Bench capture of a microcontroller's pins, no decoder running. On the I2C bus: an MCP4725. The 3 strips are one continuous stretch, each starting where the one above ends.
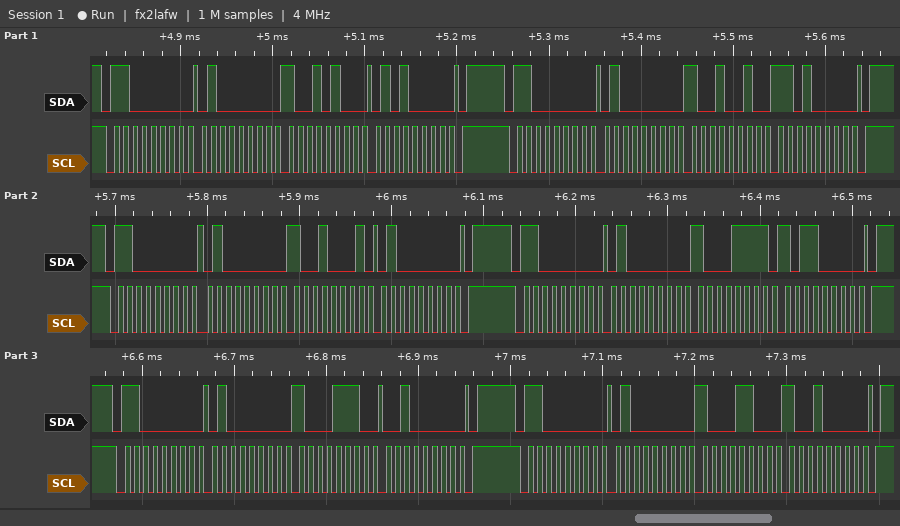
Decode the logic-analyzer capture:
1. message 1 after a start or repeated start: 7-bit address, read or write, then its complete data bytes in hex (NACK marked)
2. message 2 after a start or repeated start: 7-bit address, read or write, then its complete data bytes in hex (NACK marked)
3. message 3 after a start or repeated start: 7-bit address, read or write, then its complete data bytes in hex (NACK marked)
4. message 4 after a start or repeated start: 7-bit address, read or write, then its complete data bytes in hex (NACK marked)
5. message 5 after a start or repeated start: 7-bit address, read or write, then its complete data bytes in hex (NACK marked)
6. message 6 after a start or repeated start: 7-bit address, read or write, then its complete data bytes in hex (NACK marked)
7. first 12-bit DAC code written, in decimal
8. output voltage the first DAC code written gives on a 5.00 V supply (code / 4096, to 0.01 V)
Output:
0x60 write: 40 94 50
0x60 write: 40 92 D0
0x60 write: 40 91 40
0x60 write: 40 8F B0
0x60 write: 40 8E 20
0x60 write: 40 8C 90
2373
2.90 V
